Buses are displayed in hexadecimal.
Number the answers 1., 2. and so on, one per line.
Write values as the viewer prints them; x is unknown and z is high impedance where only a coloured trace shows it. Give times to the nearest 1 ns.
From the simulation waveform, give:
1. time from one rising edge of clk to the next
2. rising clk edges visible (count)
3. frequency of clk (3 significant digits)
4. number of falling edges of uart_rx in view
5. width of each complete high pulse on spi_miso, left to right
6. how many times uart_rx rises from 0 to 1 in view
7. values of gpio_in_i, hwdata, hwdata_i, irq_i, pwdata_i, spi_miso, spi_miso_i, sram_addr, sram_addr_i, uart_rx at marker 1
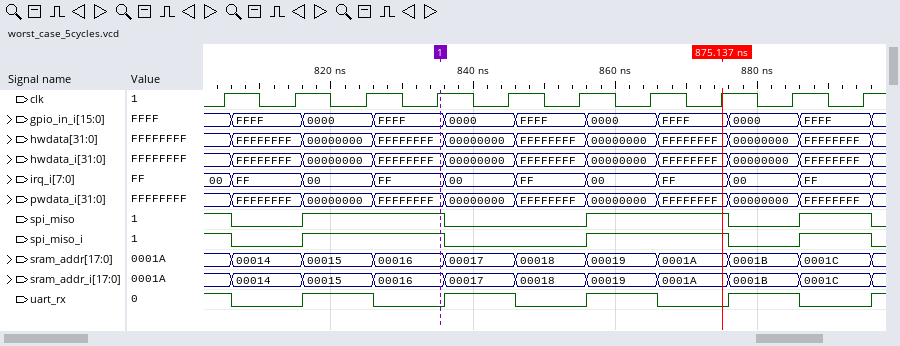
1. 10 ns
2. 10
3. 100 MHz
4. 5
5. 20 ns, 20 ns, 10 ns
6. 5
7. gpio_in_i=FFFF, hwdata=FFFFFFFF, hwdata_i=FFFFFFFF, irq_i=FF, pwdata_i=FFFFFFFF, spi_miso=1, spi_miso_i=1, sram_addr=00016, sram_addr_i=00016, uart_rx=0
